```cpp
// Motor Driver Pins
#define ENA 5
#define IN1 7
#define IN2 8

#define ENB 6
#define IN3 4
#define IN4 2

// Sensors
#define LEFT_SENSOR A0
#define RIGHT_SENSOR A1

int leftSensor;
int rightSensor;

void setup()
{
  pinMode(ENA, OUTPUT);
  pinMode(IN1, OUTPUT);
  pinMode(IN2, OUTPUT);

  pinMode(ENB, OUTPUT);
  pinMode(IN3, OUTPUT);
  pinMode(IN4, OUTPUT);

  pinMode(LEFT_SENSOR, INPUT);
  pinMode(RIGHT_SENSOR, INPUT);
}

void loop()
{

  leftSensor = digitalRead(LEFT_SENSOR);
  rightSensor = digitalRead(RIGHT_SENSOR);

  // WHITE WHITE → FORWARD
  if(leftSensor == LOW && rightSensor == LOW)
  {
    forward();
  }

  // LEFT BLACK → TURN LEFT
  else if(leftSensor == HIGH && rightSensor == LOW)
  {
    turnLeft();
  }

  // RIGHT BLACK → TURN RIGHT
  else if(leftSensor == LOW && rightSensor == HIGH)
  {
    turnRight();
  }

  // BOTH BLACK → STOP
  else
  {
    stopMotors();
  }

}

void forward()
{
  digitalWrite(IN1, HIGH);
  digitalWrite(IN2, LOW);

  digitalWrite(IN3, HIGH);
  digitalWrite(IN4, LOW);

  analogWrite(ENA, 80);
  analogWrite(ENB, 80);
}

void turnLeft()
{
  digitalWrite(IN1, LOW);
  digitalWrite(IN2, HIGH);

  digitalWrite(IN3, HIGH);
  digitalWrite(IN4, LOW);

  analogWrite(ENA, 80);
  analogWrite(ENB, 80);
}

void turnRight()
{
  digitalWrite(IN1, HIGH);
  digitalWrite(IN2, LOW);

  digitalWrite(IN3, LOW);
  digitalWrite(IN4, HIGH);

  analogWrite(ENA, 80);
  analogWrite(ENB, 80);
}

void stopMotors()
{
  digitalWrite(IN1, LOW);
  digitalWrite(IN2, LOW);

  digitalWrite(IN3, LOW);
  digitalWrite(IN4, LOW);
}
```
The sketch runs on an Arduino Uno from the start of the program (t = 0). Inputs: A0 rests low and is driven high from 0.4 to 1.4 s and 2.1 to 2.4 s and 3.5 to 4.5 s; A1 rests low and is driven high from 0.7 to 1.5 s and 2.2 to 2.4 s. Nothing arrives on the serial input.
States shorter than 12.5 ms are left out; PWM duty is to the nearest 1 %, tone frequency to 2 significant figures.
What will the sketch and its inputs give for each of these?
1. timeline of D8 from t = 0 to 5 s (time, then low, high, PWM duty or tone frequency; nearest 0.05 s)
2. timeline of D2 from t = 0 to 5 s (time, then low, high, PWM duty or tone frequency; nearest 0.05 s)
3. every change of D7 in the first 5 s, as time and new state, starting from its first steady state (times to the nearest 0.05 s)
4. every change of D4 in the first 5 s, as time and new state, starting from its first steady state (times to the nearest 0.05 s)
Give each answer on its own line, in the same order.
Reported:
0 s low; 0.4 s high; 0.7 s low; 2.1 s high; 2.2 s low; 3.5 s high; 4.5 s low
0 s low; 1.4 s high; 1.5 s low
0 s high; 0.4 s low; 1.4 s high; 2.1 s low; 2.4 s high; 3.5 s low; 4.5 s high
0 s high; 0.7 s low; 1.5 s high; 2.2 s low; 2.4 s high
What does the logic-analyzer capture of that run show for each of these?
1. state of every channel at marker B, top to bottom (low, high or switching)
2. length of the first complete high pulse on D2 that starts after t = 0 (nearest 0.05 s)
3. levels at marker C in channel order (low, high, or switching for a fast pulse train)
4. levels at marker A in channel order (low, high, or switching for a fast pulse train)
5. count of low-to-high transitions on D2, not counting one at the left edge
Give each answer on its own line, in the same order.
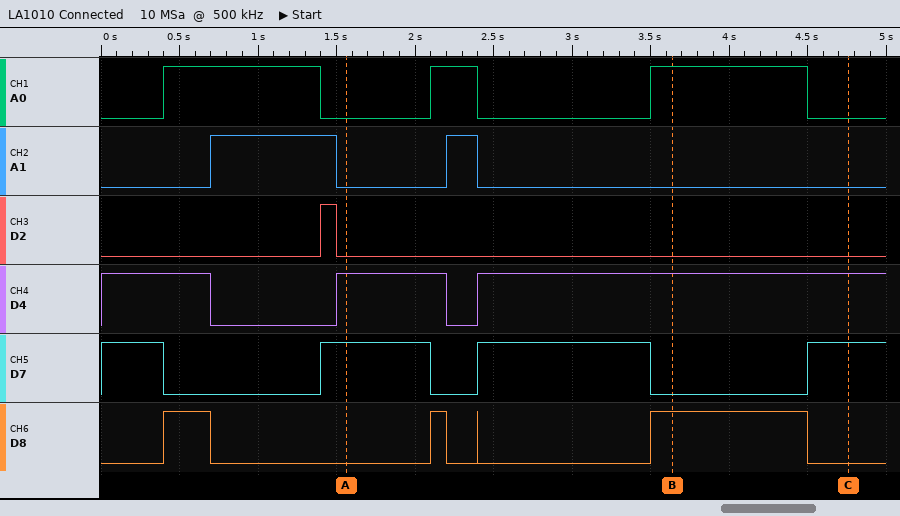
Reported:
A0 high, A1 low, D2 low, D4 high, D7 low, D8 high
0.10 s
A0 low, A1 low, D2 low, D4 high, D7 high, D8 low
A0 low, A1 low, D2 low, D4 high, D7 high, D8 low
1
